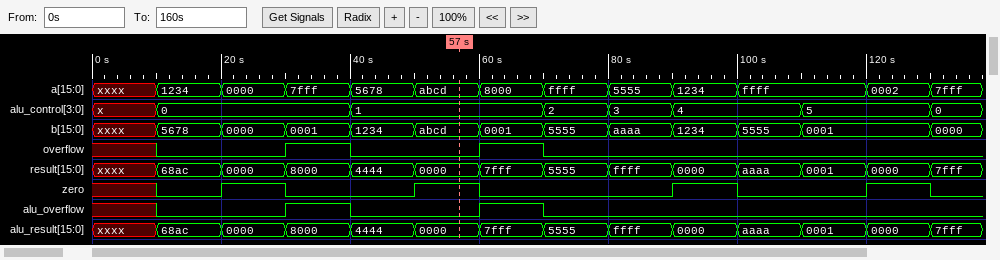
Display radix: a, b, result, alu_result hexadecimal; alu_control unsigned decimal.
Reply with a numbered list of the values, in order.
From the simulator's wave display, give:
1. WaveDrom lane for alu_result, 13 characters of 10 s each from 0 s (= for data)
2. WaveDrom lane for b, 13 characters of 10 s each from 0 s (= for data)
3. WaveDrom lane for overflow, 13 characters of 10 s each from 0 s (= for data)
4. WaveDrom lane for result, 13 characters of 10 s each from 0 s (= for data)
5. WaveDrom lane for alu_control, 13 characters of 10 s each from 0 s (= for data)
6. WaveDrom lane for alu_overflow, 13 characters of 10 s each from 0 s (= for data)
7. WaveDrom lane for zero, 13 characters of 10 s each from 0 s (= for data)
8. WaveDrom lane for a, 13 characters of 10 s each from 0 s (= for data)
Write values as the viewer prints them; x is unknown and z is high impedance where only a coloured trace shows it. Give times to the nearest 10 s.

1. {name: 'alu_result', wave: 'x============', data: '68ac 0000 8000 4444 0000 7fff 5555 ffff 0000 aaaa 0001 0000'}
2. {name: 'b', wave: 'x===========.', data: '5678 0000 0001 1234 abcd 0001 5555 aaaa 1234 5555 0001'}
3. {name: 'overflow', wave: 'x0.10.10.....'}
4. {name: 'result', wave: 'x============', data: '68ac 0000 8000 4444 0000 7fff 5555 ffff 0000 aaaa 0001 0000'}
5. {name: 'alu_control', wave: 'x=..=..===.=.', data: '0 1 2 3 4 5'}
6. {name: 'alu_overflow', wave: 'x0.10.10.....'}
7. {name: 'zero', wave: 'x010.10..10.1'}
8. {name: 'a', wave: 'x==========.=', data: '1234 0000 7fff 5678 abcd 8000 ffff 5555 1234 ffff 0002'}
